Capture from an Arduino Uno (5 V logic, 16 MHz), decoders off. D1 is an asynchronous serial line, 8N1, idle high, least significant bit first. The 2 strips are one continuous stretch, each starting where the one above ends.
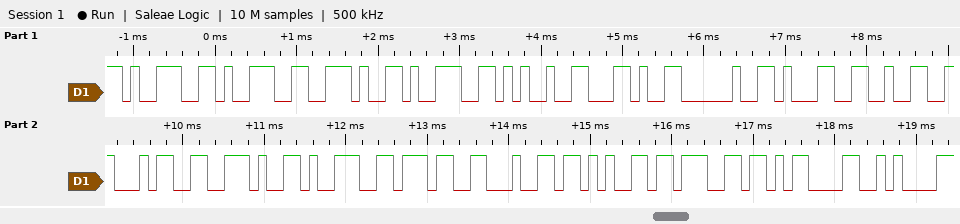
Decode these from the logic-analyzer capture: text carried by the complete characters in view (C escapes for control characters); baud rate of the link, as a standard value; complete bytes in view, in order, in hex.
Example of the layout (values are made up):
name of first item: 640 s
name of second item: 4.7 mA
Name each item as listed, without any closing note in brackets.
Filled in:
text carried by the complete characters in view: "99.9%, 124.97deg\r\n"
baud rate of the link, as a standard value: 9600 baud
complete bytes in view, in order, in hex: 39 39 2E 39 25 2C 20 31 32 34 2E 39 37 64 65 67 0D 0A
